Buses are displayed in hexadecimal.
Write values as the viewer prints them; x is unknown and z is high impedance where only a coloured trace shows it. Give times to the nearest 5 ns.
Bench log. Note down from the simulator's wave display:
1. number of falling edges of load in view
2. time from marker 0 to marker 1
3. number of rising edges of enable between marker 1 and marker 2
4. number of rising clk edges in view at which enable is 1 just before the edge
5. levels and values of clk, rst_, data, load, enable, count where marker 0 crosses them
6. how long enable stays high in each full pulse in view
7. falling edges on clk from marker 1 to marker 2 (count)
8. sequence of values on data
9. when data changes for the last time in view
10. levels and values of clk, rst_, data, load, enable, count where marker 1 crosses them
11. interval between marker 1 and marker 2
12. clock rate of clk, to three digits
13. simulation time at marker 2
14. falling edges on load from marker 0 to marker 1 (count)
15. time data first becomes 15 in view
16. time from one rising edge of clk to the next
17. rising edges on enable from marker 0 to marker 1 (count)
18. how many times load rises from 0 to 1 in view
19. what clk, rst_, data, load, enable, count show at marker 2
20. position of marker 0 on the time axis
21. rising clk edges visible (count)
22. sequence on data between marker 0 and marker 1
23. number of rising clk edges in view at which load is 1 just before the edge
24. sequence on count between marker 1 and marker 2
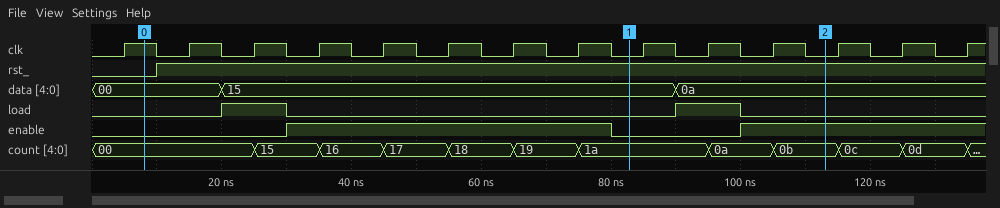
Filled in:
2
75 ns
1
9
clk=1, rst_=0, data=00, load=0, enable=0, count=00
50 ns
3
00, 15, 0a
90 ns
clk=0, rst_=1, data=15, load=0, enable=0, count=1a
30 ns
100 MHz
115 ns
1
20 ns
10 ns
1
2
clk=0, rst_=1, data=0a, load=0, enable=1, count=0b
10 ns
14
00, 15
2
1a, 0a, 0b
